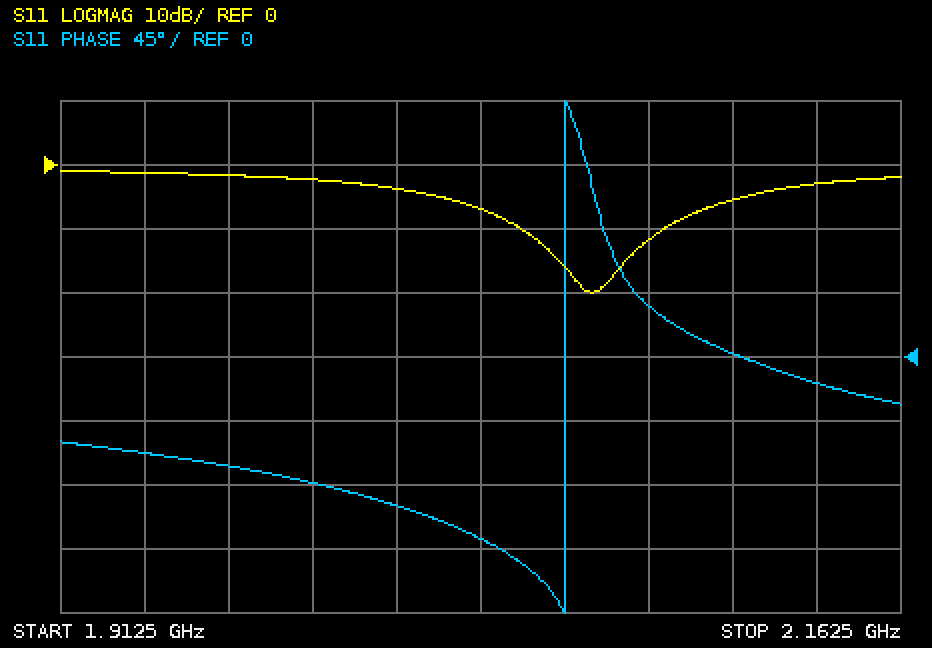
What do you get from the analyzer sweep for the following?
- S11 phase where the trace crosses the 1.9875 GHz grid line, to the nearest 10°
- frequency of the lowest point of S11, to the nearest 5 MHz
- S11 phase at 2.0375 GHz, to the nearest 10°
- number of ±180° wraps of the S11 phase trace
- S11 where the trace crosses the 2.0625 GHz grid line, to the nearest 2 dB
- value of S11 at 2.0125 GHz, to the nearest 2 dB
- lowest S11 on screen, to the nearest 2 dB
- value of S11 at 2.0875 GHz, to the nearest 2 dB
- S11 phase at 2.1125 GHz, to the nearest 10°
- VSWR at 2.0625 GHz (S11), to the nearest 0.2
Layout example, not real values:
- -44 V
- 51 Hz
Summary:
- -90°
- 2.070 GHz
- -130°
- 1
- -16 dB
- -4 dB
- -20 dB
- -12 dB
- 0°
- 1.4
